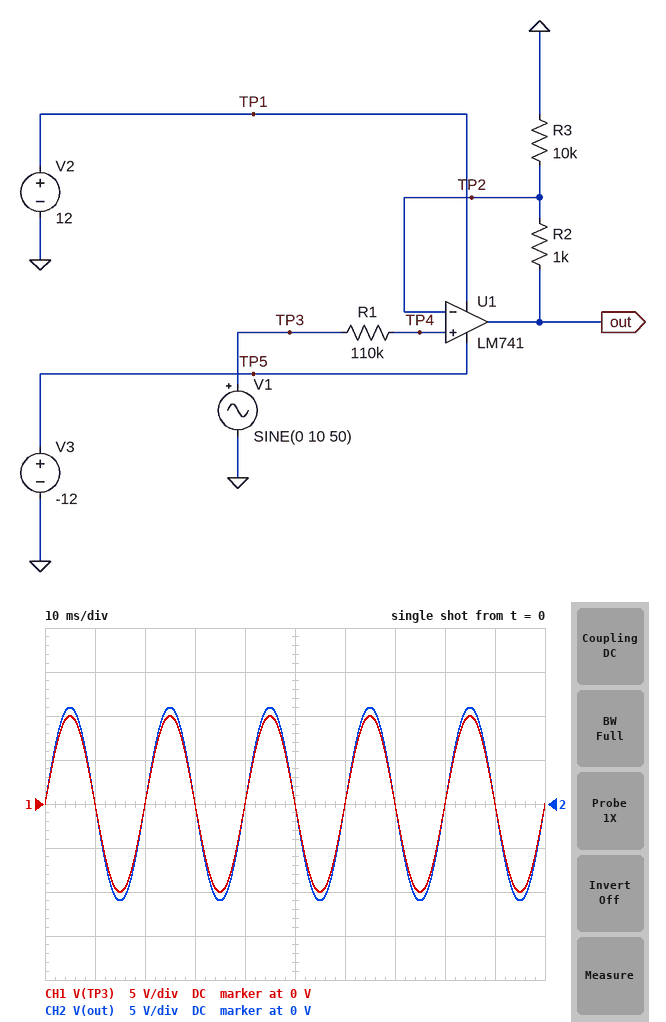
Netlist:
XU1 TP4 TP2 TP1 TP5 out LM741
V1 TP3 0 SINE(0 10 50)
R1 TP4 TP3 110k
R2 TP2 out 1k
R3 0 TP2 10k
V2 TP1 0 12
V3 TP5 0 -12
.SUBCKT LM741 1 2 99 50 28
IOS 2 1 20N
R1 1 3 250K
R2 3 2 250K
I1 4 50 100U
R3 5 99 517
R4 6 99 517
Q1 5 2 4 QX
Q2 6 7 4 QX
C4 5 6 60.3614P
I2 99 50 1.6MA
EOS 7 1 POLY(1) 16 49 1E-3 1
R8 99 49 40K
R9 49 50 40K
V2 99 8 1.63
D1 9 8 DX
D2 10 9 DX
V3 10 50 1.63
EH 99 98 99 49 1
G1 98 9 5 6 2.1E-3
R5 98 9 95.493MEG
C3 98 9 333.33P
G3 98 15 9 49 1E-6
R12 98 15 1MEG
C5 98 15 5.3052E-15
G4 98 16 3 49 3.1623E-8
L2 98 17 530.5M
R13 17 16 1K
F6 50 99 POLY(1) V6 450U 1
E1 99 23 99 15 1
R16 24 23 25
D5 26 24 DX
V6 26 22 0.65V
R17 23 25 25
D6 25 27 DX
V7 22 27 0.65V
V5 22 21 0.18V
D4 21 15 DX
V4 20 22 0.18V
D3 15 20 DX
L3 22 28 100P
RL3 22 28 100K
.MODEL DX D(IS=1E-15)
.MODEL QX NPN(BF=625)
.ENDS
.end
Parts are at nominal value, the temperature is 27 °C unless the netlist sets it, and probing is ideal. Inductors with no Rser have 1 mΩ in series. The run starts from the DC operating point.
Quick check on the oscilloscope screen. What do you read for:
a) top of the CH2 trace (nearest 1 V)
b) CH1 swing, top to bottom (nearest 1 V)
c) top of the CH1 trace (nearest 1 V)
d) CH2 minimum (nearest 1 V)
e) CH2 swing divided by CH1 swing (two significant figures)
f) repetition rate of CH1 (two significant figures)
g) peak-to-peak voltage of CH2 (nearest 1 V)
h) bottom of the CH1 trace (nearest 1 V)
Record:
11 V
20 V
10 V
-11 V
1.1
50 Hz
22 V
-10 V
